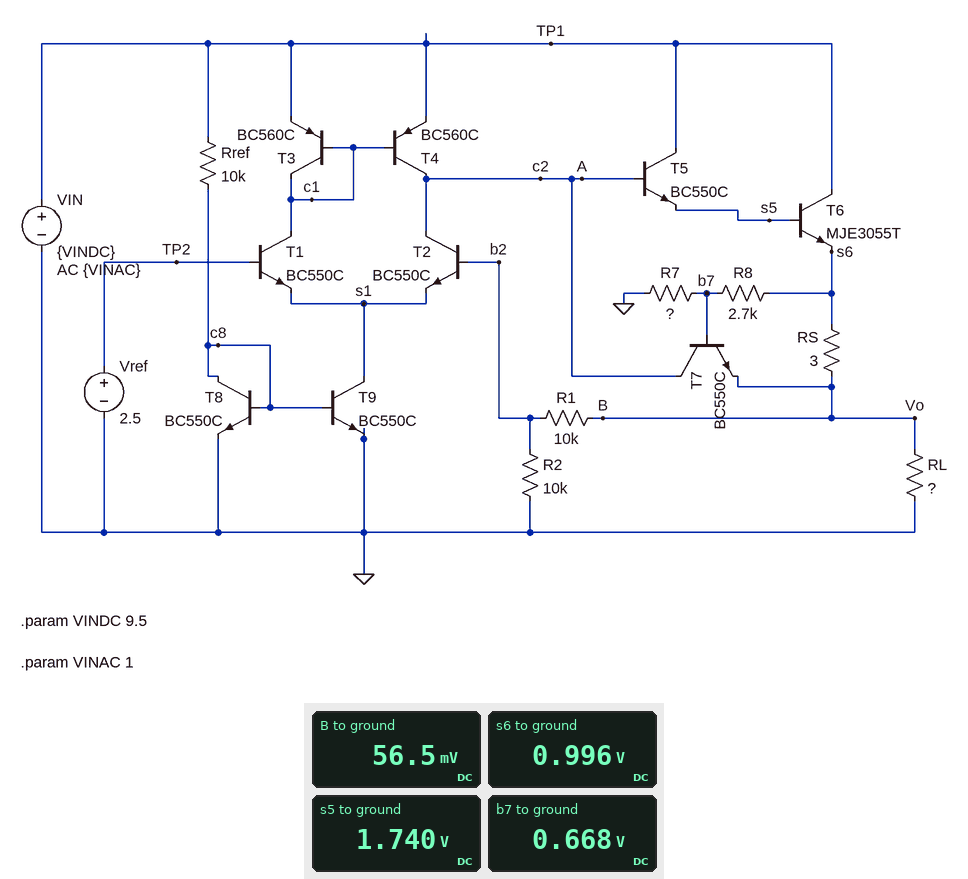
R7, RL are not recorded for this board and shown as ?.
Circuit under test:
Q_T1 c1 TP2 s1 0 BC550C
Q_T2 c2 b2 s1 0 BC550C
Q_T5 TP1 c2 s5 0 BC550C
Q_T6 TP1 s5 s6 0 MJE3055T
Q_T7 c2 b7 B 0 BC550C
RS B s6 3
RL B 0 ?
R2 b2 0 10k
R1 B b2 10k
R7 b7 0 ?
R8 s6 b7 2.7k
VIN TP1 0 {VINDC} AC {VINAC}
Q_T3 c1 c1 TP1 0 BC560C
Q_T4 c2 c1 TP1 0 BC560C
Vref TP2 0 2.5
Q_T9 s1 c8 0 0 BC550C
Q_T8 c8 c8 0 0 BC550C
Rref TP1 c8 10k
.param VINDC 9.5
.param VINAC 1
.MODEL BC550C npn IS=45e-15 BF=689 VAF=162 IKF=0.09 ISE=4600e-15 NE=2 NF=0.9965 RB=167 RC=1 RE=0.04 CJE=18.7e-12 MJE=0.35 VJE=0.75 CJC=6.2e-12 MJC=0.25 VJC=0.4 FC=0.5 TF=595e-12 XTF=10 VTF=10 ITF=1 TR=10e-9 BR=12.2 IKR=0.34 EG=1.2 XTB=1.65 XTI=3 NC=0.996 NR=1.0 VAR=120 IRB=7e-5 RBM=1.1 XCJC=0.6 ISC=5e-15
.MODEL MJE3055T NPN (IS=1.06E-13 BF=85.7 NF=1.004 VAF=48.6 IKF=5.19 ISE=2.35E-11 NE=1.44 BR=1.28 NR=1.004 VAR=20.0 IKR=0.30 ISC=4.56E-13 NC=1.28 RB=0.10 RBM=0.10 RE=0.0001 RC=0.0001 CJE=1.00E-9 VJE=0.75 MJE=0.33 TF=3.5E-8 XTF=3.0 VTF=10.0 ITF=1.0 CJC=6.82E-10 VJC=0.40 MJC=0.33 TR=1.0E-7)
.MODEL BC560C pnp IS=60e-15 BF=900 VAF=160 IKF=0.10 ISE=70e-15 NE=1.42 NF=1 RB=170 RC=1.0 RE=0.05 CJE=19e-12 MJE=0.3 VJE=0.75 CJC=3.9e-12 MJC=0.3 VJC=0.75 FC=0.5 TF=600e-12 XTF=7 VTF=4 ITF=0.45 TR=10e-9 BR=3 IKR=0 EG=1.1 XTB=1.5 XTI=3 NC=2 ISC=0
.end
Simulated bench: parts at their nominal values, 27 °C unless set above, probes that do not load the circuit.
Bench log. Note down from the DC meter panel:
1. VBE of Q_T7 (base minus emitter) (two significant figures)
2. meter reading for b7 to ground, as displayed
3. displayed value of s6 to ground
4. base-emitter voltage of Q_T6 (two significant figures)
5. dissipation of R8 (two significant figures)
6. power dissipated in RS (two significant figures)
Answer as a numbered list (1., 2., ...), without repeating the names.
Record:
1. 610 mV
2. 0.668 V
3. 0.996 V
4. 740 mV
5. 40 µW
6. 290 mW
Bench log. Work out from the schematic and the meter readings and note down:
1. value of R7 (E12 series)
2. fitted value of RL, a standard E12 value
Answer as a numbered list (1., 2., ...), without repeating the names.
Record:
1. 5.6 kΩ
2. 0.18 Ω
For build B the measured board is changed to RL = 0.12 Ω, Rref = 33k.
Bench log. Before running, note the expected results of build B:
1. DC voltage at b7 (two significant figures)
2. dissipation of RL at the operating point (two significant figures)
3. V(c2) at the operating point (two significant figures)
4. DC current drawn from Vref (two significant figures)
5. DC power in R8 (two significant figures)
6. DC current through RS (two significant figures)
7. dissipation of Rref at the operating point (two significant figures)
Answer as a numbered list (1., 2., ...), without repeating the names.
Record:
1. 610 mV
2. 10 mW
3. 2.3 V
4. 720 nA
5. 33 µW
6. 290 mA
7. 2.4 mW
